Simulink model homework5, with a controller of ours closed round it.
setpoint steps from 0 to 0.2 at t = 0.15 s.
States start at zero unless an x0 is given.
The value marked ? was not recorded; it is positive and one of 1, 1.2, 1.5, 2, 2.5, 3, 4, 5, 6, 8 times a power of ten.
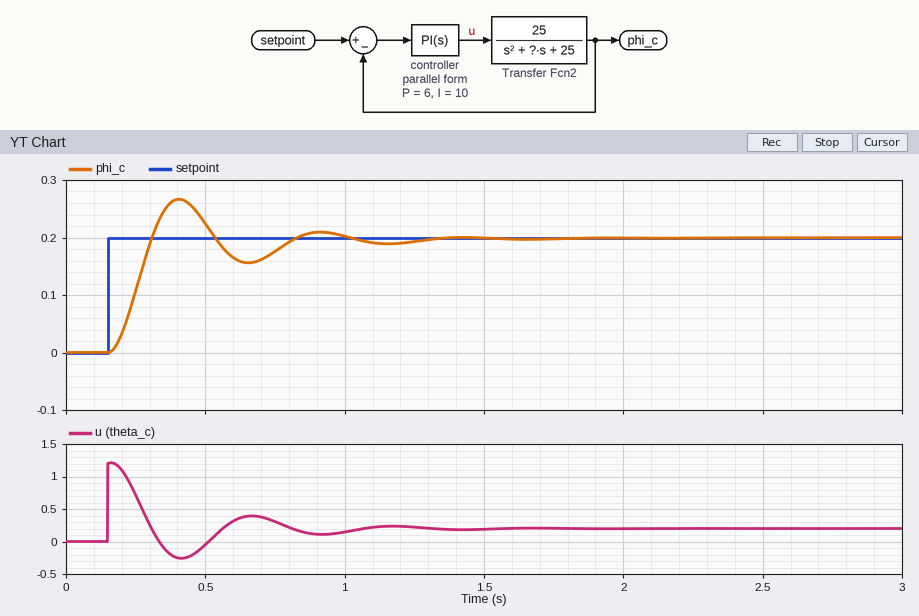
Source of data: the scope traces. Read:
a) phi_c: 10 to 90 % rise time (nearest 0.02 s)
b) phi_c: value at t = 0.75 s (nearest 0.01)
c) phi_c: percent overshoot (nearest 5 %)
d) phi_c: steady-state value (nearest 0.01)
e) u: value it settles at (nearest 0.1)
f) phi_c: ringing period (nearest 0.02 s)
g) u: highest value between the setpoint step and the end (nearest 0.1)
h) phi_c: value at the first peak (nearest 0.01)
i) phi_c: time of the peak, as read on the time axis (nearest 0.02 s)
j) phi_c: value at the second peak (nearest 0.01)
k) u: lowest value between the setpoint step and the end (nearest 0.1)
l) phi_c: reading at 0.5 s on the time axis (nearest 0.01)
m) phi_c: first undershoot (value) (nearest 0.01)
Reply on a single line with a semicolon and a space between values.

0.10 s; 0.18; 35 %; 0.20; 0.2; 0.50 s; 1.2; 0.27; 0.40 s; 0.21; -0.3; 0.22; 0.16
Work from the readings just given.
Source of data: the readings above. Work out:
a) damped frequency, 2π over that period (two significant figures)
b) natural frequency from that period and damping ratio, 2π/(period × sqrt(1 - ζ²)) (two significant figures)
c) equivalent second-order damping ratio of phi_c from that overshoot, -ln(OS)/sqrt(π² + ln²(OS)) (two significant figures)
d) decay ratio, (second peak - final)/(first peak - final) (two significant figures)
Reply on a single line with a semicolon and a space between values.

13 rad/s; 13 rad/s; 0.32; 0.14
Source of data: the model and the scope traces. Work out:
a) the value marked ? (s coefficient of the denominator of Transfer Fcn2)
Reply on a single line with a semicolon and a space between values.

8
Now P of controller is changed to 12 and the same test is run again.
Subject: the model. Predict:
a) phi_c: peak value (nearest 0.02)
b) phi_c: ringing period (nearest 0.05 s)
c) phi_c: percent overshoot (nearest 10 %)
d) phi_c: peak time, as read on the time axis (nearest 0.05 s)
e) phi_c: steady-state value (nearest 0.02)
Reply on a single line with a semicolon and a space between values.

0.28; 0.35 s; 40 %; 0.35 s; 0.20
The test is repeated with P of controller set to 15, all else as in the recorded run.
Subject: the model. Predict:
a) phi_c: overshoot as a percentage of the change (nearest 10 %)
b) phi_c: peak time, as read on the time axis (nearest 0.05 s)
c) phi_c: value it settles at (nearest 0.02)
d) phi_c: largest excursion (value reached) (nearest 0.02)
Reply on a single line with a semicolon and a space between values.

50 %; 0.30 s; 0.20; 0.30
